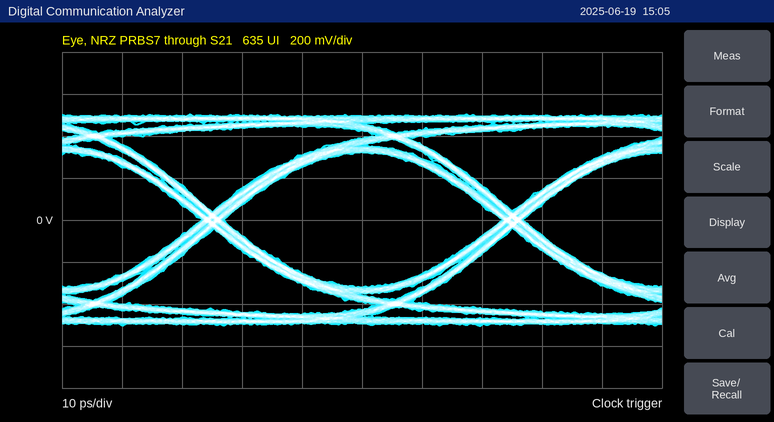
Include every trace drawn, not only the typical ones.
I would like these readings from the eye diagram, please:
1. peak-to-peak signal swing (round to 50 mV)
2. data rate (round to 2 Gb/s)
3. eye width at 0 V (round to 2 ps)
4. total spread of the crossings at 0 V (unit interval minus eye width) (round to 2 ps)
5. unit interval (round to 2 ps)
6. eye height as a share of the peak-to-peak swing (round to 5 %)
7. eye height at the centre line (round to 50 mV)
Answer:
1.00 V
20 Gb/s
46 ps
4 ps
50 ps
65 %
650 mV
